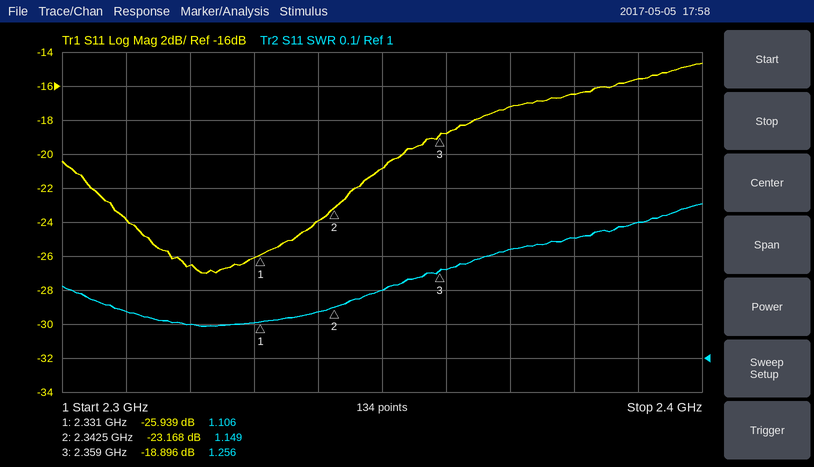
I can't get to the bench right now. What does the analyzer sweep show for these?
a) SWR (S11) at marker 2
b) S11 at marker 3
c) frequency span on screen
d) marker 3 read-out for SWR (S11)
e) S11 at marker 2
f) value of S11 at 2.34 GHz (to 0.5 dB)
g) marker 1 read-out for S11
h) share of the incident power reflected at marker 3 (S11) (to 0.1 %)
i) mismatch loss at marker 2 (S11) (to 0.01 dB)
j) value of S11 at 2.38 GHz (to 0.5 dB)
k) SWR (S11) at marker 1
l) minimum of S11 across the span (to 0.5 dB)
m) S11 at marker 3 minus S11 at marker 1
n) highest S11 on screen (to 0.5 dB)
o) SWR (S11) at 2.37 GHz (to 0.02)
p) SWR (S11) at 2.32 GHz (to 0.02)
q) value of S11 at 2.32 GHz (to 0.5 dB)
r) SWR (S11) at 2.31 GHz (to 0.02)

1.149
-18.896 dB
100 MHz
1.256
-23.168 dB
-24.0 dB
-25.939 dB
1.3 %
0.02 dB
-16.5 dB
1.106
-27.0 dB
7.043 dB
-14.5 dB
1.32
1.10
-26.5 dB
1.14
